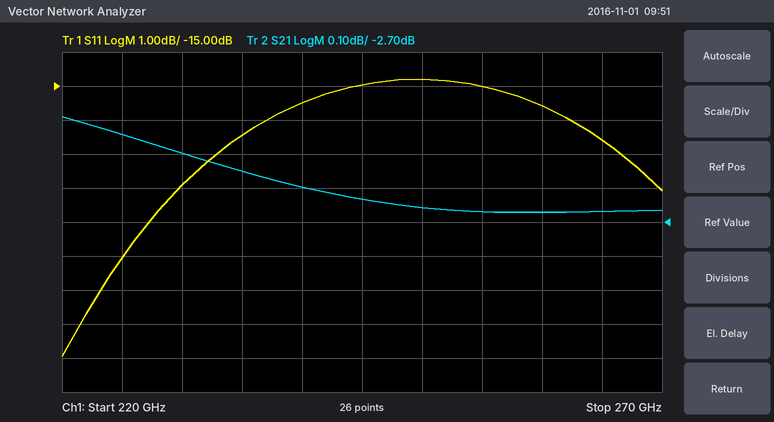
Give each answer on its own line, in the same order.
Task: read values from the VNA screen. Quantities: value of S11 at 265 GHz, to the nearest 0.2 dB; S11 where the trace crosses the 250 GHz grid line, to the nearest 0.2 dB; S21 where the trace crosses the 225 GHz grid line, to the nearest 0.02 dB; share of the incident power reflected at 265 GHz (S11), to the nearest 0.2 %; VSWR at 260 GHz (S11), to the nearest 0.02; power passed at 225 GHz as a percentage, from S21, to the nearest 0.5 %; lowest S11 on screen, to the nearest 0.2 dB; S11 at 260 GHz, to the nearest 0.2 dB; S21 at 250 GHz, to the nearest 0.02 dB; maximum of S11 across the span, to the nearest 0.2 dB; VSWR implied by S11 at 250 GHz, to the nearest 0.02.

-16.6 dB
-14.8 dB
-2.44 dB
2.2 %
1.40
57.0 %
-23.0 dB
-15.6 dB
-2.66 dB
-14.8 dB
1.44
